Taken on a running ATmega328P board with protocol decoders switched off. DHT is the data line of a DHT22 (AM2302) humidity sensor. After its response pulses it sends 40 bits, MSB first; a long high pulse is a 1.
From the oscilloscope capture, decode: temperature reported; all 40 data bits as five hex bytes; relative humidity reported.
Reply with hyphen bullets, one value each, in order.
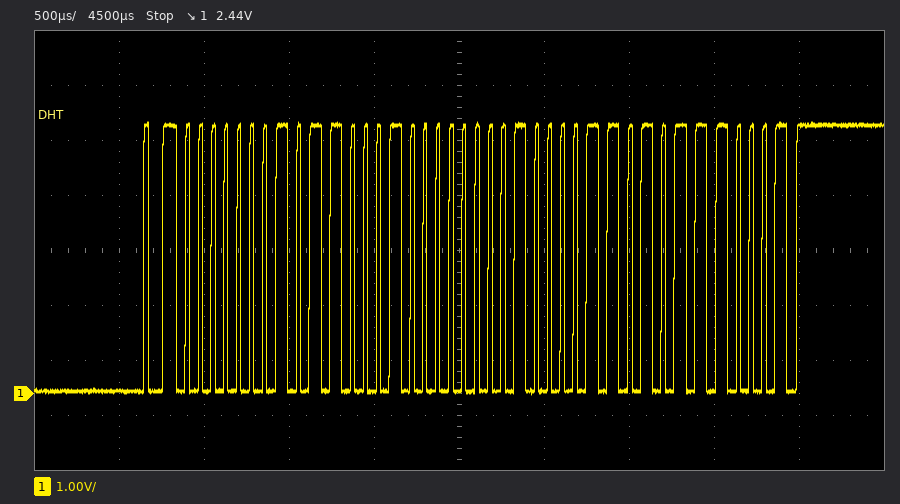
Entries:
- 26.9 °C
- 01 62 01 0D 71
- 35.4 %
